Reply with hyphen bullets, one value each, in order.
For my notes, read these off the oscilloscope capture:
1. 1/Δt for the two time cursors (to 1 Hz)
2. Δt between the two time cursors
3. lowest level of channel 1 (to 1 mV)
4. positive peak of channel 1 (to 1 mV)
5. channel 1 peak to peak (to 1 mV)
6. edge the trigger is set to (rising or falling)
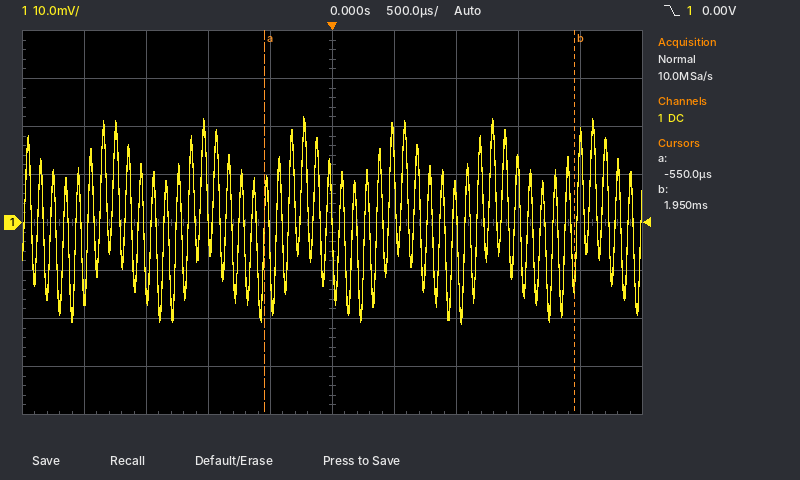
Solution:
- 400 Hz
- 2.50 ms
- -21 mV
- 22 mV
- 43 mV
- falling
